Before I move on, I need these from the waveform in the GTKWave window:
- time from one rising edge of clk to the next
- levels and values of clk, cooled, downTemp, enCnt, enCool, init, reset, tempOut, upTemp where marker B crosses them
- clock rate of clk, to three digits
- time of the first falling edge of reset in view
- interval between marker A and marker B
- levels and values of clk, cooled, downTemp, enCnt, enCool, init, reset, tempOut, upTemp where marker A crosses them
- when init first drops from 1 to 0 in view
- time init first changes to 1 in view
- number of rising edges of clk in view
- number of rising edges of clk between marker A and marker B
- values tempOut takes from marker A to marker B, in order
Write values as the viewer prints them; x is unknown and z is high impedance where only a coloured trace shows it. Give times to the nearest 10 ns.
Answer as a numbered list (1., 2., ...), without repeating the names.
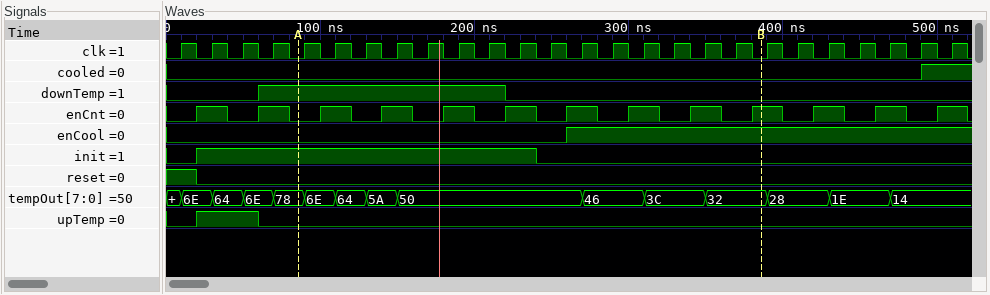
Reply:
1. 20 ns
2. clk=0, cooled=0, downTemp=0, enCnt=1, enCool=1, init=0, reset=0, tempOut=32, upTemp=0
3. 50.0 MHz
4. 20 ns
5. 300 ns
6. clk=0, cooled=0, downTemp=1, enCnt=0, enCool=0, init=1, reset=0, tempOut=78, upTemp=0
7. 240 ns
8. 20 ns
9. 26
10. 15
11. 78, 6E, 64, 5A, 50, 46, 3C, 32
